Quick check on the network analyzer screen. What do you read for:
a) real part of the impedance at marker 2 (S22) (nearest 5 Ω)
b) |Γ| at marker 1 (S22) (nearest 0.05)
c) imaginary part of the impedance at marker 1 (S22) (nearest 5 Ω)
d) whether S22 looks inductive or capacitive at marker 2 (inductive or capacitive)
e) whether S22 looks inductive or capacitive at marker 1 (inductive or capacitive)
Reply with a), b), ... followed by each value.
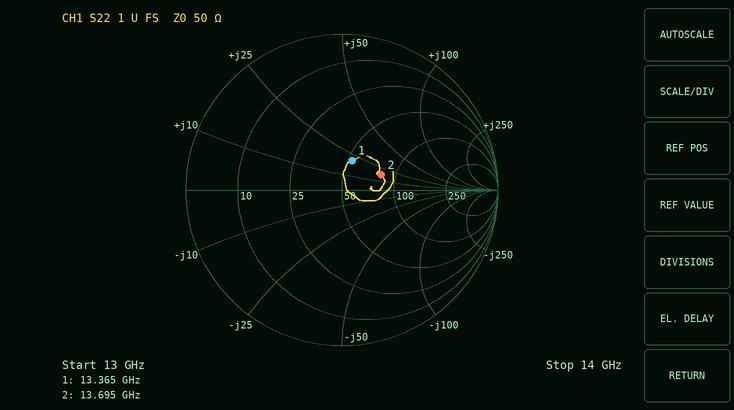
a) 80 Ω
b) 0.20
c) +20 Ω
d) inductive
e) inductive
